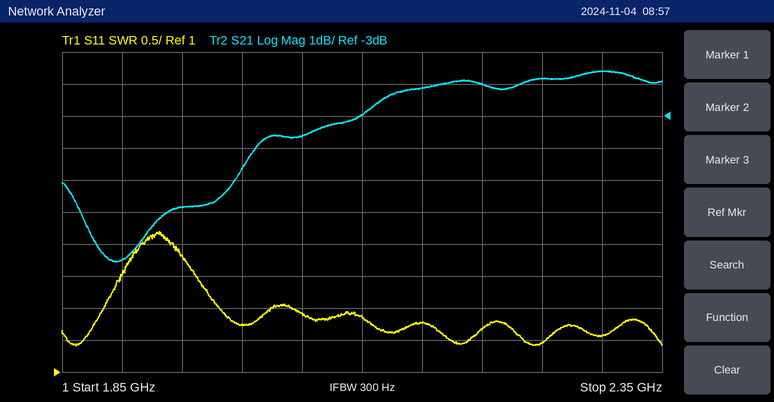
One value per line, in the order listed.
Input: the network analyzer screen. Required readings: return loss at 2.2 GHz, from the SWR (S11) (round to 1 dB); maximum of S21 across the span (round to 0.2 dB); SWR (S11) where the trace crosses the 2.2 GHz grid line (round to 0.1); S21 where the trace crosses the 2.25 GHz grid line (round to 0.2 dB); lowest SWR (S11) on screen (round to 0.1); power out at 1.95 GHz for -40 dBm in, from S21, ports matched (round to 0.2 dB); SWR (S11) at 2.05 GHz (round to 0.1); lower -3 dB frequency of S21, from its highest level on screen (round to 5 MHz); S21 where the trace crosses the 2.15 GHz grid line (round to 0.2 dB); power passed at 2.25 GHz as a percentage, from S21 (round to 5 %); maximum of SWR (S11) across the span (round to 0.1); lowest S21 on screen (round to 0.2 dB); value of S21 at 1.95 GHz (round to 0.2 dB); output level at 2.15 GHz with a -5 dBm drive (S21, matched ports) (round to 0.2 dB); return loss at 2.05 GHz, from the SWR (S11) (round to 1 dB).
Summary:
12 dB
-1.6 dB
1.7
-1.8 dB
1.4
-45.8 dBm
1.9
2.000 GHz
-2.2 dB
65 %
3.2
-7.6 dB
-5.8 dB
-7.2 dBm
10 dB
